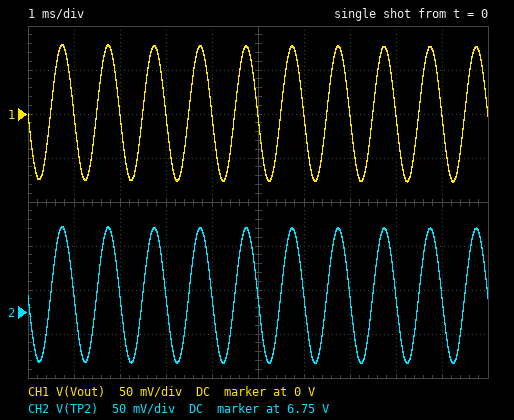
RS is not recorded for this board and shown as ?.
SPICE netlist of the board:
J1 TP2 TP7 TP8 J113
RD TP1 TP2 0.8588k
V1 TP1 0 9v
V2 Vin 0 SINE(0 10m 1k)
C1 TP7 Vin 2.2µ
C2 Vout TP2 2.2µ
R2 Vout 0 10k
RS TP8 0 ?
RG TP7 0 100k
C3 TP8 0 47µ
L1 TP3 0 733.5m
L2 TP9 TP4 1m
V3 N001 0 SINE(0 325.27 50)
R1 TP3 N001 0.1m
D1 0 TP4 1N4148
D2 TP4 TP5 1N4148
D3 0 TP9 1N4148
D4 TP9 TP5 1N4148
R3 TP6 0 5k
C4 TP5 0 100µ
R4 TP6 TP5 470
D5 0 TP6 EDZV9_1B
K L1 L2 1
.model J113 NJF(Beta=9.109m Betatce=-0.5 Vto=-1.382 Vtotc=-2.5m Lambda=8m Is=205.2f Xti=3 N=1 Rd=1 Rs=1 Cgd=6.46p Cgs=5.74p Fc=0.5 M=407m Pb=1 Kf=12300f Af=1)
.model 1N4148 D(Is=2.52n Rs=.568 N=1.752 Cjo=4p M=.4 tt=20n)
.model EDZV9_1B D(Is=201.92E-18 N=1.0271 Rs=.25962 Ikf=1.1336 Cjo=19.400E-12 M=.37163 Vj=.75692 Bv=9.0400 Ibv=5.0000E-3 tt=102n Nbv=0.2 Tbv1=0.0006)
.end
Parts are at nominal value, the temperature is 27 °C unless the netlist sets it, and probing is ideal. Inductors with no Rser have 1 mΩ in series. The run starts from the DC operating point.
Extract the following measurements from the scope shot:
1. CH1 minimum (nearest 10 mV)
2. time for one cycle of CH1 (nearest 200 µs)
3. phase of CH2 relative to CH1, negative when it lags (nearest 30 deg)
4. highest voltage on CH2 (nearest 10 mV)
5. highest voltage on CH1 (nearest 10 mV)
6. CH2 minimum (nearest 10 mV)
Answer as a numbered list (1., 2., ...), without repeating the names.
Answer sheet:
1. -80 mV
2. 1.0 ms
3. 0 deg
4. 6.85 V
5. 80 mV
6. 6.69 V
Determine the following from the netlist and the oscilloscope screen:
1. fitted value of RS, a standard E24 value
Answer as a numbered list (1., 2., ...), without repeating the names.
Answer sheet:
1. 330 Ω
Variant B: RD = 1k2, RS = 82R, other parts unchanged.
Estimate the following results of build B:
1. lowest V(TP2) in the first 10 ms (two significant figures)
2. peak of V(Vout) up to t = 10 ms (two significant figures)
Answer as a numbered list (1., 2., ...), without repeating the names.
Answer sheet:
1. 1.2 V
2. 53 mV
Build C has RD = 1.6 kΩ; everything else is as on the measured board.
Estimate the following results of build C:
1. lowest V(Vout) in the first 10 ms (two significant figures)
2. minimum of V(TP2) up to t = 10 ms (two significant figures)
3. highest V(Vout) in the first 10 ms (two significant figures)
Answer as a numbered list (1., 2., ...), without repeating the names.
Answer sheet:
1. -130 mV
2. 4.7 V
3. 130 mV
